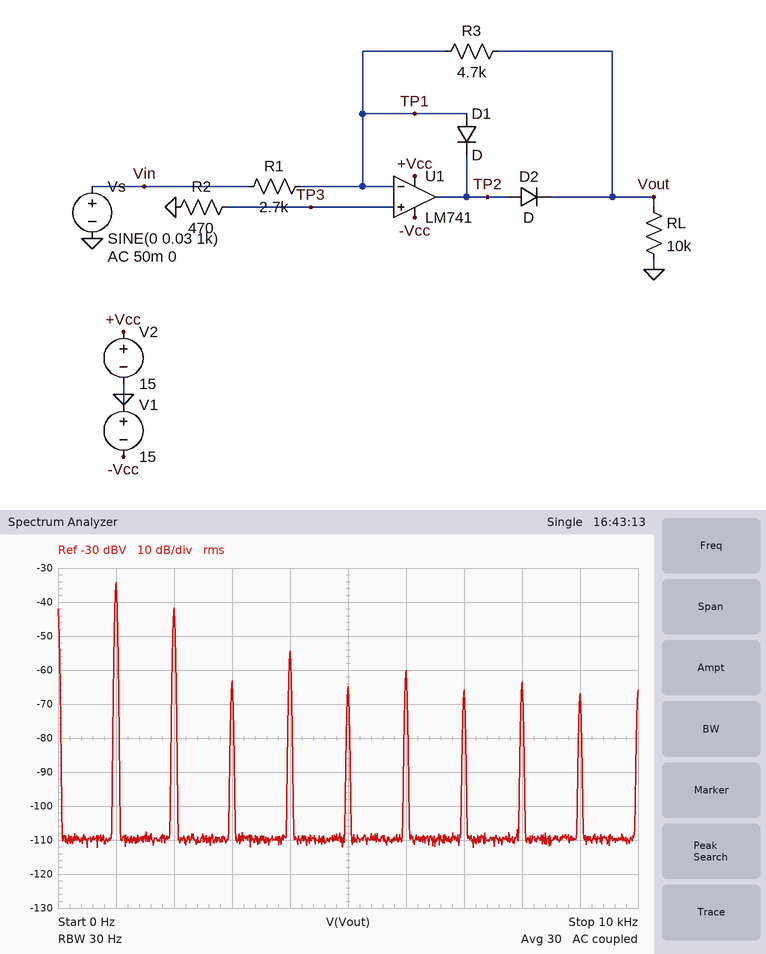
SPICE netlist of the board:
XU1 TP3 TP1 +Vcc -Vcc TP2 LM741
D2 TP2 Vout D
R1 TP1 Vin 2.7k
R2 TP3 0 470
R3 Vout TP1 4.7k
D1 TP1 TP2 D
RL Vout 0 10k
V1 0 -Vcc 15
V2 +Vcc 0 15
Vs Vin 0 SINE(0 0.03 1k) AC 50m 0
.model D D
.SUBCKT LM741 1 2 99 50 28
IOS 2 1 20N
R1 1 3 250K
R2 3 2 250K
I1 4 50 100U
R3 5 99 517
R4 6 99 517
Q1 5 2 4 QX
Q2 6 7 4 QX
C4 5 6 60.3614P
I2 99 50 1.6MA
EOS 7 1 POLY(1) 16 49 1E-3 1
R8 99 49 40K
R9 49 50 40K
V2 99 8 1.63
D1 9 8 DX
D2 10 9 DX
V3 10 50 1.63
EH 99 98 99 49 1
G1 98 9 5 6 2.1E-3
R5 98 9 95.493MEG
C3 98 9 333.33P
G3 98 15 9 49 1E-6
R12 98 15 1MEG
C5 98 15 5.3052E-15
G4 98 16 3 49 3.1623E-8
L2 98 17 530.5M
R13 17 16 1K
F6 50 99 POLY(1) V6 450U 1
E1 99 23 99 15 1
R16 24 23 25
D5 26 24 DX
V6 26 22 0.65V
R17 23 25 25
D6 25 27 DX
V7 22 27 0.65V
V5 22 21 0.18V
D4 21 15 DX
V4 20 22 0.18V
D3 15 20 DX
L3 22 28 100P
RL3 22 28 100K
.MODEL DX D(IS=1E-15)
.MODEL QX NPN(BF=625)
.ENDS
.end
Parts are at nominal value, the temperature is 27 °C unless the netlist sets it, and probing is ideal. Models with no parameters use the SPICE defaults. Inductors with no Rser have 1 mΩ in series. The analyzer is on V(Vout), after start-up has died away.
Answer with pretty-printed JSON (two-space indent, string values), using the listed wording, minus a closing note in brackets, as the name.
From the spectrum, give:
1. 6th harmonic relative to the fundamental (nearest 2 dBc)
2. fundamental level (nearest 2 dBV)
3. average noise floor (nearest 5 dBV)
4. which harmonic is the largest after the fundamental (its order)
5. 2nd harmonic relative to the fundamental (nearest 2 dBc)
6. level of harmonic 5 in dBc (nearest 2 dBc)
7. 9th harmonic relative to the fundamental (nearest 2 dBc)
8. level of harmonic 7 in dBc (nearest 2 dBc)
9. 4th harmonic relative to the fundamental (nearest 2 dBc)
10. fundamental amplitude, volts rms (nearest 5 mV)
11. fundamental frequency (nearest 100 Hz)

{
  "6th harmonic relative to the fundamental": "-26 dBc",
  "fundamental level": "-34 dBV",
  "average noise floor": "-110 dBV",
  "which harmonic is the largest after the fundamental": "2",
  "2nd harmonic relative to the fundamental": "-8 dBc",
  "level of harmonic 5 in dBc": "-30 dBc",
  "9th harmonic relative to the fundamental": "-32 dBc",
  "level of harmonic 7 in dBc": "-32 dBc",
  "4th harmonic relative to the fundamental": "-20 dBc",
  "fundamental amplitude, volts rms": "20 mV",
  "fundamental frequency": "1.0 kHz"
}
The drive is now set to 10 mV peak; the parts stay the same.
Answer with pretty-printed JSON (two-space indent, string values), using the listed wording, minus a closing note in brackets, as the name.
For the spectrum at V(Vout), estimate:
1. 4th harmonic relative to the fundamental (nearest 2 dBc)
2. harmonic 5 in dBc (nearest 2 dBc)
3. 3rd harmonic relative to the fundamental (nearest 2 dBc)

{
  "4th harmonic relative to the fundamental": "-18 dBc",
  "harmonic 5 in dBc": "-26 dBc",
  "3rd harmonic relative to the fundamental": "-22 dBc"
}
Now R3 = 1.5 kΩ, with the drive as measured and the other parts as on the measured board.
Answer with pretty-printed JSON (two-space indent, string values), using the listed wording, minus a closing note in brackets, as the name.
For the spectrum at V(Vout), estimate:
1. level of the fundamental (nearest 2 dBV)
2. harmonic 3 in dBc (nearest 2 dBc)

{
  "level of the fundamental": "-44 dBV",
  "harmonic 3 in dBc": "-22 dBc"
}
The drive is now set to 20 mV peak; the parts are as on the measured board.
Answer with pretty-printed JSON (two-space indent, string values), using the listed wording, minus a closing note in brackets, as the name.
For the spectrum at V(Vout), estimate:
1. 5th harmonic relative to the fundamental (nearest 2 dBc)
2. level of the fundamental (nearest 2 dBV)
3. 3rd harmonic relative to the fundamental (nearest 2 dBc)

{
  "5th harmonic relative to the fundamental": "-28 dBc",
  "level of the fundamental": "-38 dBV",
  "3rd harmonic relative to the fundamental": "-26 dBc"
}
